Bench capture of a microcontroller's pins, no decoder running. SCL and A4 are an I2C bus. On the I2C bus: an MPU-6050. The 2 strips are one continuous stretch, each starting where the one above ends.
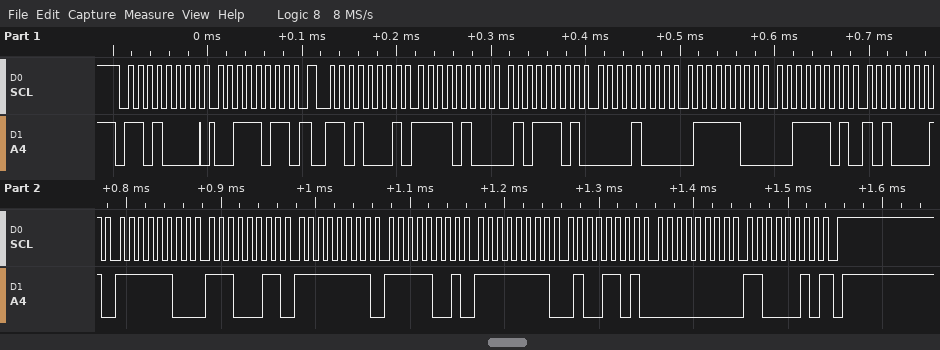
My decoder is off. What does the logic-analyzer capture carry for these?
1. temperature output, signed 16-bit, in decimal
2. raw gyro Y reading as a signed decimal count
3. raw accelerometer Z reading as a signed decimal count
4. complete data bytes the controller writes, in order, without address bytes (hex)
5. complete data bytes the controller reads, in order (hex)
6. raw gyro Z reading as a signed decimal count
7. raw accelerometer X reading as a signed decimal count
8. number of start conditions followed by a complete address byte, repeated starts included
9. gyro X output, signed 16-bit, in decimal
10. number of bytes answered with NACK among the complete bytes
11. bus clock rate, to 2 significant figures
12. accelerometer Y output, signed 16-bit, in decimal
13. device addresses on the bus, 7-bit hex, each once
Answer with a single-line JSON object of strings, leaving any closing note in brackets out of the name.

{"temperature output, signed 16-bit, in decimal": "-797", "raw gyro Y reading as a signed decimal count": "-179", "raw accelerometer Z reading as a signed decimal count": "15777", "complete data bytes the controller writes, in order, without address bytes": "3B", "complete data bytes the controller reads, in order": "F4 5D 08 7C 3D A1 FC E3 FF F9 FF 4D 00 C2", "raw gyro Z reading as a signed decimal count": "194", "raw accelerometer X reading as a signed decimal count": "-2979", "number of start conditions followed by a complete address byte, repeated starts included": "2", "gyro X output, signed 16-bit, in decimal": "-7", "number of bytes answered with NACK among the complete bytes": "1", "bus clock rate, to 2 significant figures": "100 kHz", "accelerometer Y output, signed 16-bit, in decimal": "2172", "device addresses on the bus, 7-bit hex, each once": "0x68"}
